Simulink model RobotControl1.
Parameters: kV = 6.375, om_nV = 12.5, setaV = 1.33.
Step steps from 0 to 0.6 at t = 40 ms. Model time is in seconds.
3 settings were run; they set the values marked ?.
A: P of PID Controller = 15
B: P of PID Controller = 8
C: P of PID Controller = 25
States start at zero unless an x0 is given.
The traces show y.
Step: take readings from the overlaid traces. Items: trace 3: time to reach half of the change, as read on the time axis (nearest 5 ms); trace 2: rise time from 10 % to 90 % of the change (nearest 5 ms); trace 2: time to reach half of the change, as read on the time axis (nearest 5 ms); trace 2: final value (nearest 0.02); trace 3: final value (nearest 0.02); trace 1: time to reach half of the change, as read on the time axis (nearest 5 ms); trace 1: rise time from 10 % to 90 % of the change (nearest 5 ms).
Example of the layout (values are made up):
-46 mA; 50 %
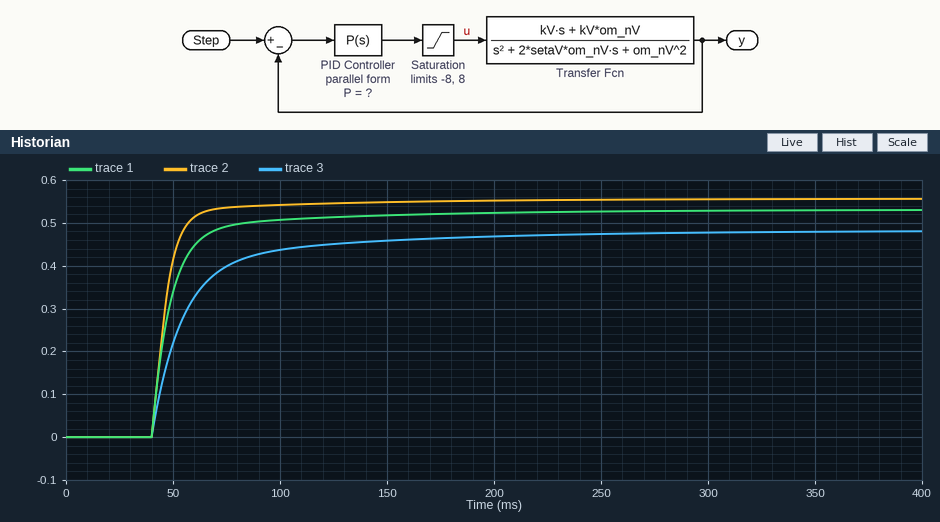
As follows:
50 ms; 15 ms; 45 ms; 0.56; 0.48; 45 ms; 25 ms
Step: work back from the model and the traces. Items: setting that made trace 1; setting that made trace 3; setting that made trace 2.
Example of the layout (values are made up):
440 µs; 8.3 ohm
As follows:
A; B; C
